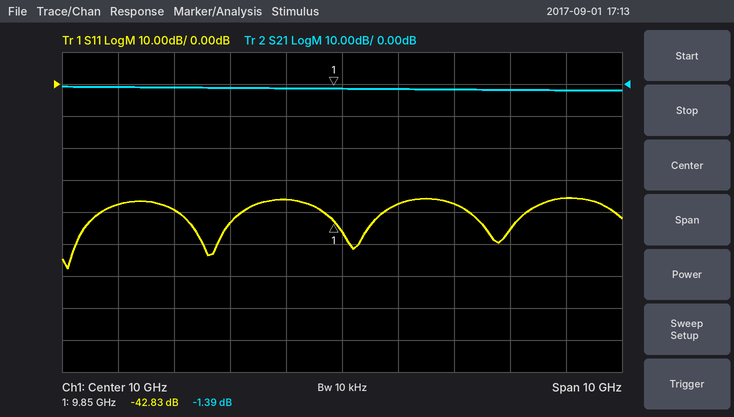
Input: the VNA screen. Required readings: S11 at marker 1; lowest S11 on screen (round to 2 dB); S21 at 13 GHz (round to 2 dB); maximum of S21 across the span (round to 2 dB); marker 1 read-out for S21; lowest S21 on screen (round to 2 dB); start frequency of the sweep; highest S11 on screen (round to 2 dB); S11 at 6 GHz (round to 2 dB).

-42.83 dB
-58 dB
-2 dB
0 dB
-1.39 dB
-2 dB
5 GHz
-36 dB
-38 dB
